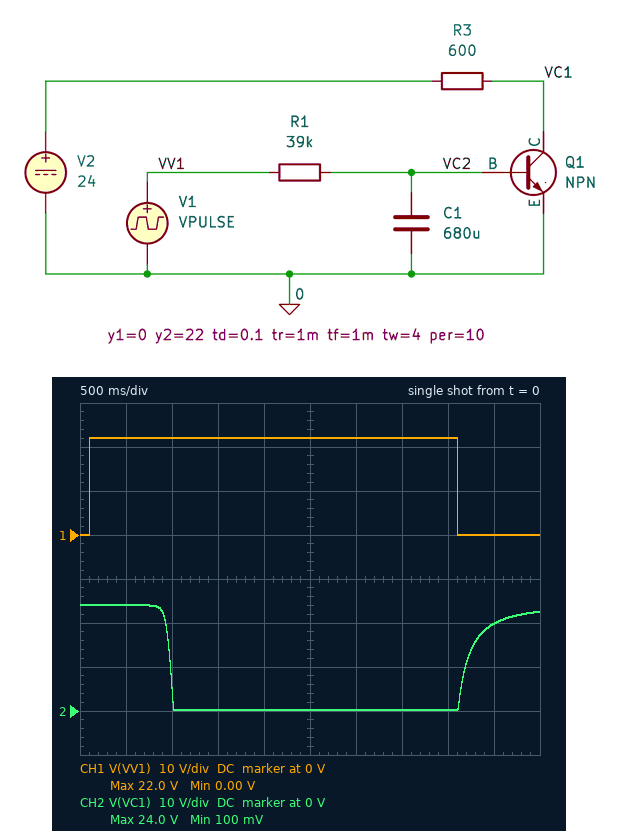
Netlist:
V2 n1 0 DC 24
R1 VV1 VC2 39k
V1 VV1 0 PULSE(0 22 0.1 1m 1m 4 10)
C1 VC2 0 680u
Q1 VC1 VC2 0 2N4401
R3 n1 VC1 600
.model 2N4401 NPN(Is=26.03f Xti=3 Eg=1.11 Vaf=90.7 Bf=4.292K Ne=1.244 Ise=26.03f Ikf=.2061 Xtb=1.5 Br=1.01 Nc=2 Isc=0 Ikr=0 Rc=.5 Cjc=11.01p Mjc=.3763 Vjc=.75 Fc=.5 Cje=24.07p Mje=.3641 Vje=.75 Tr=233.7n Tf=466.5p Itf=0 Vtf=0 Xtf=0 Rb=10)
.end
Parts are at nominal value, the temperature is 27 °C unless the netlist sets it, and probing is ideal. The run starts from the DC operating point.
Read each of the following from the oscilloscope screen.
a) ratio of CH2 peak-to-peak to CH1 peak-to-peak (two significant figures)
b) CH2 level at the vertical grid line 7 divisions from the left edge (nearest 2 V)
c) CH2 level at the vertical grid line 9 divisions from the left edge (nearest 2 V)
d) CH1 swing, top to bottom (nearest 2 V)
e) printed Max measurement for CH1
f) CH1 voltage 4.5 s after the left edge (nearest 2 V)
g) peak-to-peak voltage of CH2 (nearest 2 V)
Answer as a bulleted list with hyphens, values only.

- 1.1
- 0 V
- 20 V
- 22 V
- 22.0 V
- 0 V
- 24 V
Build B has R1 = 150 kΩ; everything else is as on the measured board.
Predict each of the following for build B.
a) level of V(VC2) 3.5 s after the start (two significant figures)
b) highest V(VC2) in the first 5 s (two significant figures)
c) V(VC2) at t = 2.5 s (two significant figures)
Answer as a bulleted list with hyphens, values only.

- 700 mV
- 720 mV
- 510 mV
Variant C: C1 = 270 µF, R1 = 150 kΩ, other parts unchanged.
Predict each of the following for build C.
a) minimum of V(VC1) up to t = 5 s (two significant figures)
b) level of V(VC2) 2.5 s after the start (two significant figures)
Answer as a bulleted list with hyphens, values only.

- 6.3 V
- 720 mV
